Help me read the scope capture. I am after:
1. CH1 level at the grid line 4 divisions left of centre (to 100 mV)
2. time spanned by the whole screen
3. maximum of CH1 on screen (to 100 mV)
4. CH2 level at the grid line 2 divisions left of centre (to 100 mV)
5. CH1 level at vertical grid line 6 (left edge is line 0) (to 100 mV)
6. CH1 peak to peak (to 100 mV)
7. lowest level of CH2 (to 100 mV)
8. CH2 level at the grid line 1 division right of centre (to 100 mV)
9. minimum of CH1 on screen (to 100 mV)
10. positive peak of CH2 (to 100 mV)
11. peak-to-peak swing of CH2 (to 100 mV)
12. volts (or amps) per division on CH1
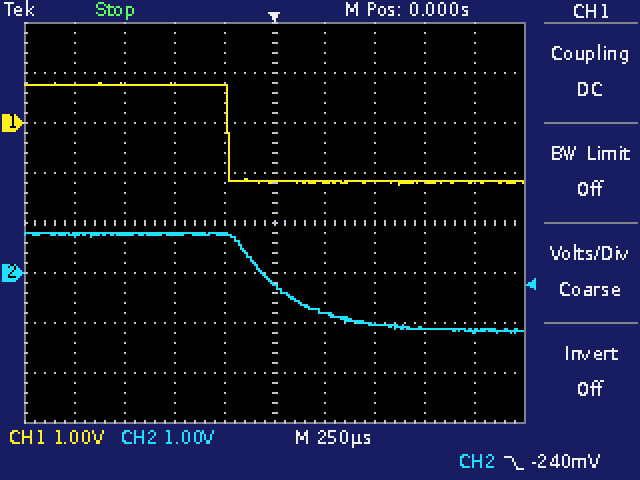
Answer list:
800 mV
2.5 ms
800 mV
800 mV
-1.2 V
2.0 V
-1.2 V
-800 mV
-1.2 V
800 mV
2.0 V
1 V
